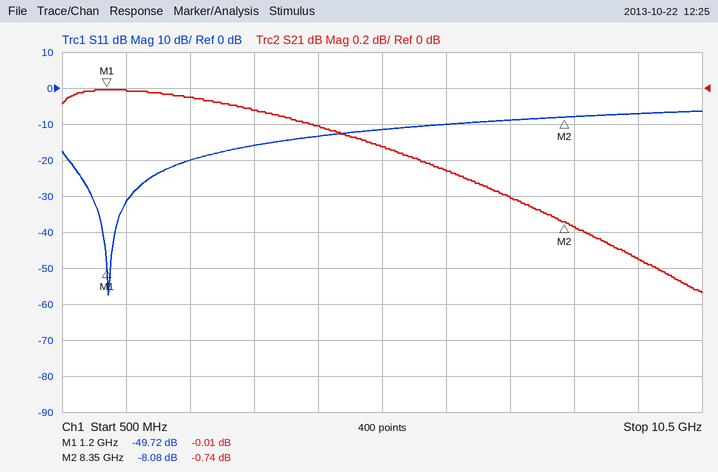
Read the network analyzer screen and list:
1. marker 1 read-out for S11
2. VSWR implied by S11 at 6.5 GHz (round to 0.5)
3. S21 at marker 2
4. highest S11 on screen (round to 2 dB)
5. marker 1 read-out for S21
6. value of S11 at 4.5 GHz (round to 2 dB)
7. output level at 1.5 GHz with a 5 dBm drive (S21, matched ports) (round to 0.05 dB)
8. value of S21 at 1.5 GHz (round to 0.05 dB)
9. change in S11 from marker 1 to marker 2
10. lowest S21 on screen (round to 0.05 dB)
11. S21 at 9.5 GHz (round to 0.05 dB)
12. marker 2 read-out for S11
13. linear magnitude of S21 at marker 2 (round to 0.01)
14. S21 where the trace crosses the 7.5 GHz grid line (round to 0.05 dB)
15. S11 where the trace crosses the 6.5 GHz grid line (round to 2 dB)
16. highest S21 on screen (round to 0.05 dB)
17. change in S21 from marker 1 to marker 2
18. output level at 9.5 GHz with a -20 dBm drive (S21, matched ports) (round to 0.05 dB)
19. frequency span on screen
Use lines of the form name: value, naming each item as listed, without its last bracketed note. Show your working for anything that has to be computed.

marker 1 read-out for S11: -49.72 dB
VSWR implied by S11 at 6.5 GHz: |Γ| = 10^(-10/20) = 0.3162; VSWR = (1 + 0.3162)/(1 − 0.3162) ≈ 1.92, so 2.0 to the nearest 0.5
S21 at marker 2: -0.74 dB
highest S11 on screen: -6 dB
marker 1 read-out for S21: -0.01 dB
value of S11 at 4.5 GHz: -14 dB
output level at 1.5 GHz with a 5 dBm drive (S21, matched ports): 5 dBm + (0.00 dB) = 5.00 dBm
value of S21 at 1.5 GHz: 0.00 dB
change in S11 from marker 1 to marker 2: -8.08 − (-49.72) = 41.64 dB
lowest S21 on screen: -1.15 dB
S21 at 9.5 GHz: -0.95 dB
marker 2 read-out for S11: -8.08 dB
linear magnitude of S21 at marker 2: 10^(-0.74/20) ≈ 0.92
S21 where the trace crosses the 7.5 GHz grid line: -0.60 dB
S11 where the trace crosses the 6.5 GHz grid line: -10 dB
highest S21 on screen: 0.00 dB
change in S21 from marker 1 to marker 2: -0.74 − (-0.01) = -0.73 dB
output level at 9.5 GHz with a -20 dBm drive (S21, matched ports): -20 dBm + (-0.95 dB) = -20.95 dBm
frequency span on screen: 10 GHz
